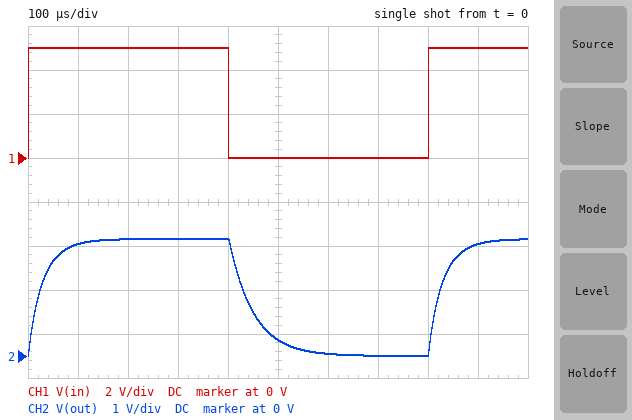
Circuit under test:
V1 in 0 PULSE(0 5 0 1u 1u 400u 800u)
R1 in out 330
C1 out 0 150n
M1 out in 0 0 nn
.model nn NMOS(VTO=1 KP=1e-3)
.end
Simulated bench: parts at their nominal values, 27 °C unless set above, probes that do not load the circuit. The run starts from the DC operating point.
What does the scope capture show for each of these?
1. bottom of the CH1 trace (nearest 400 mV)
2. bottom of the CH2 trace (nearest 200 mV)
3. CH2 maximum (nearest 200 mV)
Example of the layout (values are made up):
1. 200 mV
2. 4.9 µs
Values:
1. 0 V
2. 0 V
3. 2.6 V
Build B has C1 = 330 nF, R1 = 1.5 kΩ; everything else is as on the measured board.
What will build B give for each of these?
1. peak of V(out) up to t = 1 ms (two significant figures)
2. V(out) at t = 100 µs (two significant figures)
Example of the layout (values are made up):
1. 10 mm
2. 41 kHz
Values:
1. 770 mV
2. 550 mV
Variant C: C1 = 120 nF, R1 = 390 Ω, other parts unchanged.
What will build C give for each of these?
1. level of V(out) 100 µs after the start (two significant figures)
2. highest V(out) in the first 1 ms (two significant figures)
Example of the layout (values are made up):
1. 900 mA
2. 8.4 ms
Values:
1. 2.3 V
2. 2.4 V
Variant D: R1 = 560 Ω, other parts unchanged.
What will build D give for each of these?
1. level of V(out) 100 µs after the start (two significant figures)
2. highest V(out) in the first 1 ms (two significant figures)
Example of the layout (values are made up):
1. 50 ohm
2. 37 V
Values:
1. 1.7 V
2. 1.8 V
